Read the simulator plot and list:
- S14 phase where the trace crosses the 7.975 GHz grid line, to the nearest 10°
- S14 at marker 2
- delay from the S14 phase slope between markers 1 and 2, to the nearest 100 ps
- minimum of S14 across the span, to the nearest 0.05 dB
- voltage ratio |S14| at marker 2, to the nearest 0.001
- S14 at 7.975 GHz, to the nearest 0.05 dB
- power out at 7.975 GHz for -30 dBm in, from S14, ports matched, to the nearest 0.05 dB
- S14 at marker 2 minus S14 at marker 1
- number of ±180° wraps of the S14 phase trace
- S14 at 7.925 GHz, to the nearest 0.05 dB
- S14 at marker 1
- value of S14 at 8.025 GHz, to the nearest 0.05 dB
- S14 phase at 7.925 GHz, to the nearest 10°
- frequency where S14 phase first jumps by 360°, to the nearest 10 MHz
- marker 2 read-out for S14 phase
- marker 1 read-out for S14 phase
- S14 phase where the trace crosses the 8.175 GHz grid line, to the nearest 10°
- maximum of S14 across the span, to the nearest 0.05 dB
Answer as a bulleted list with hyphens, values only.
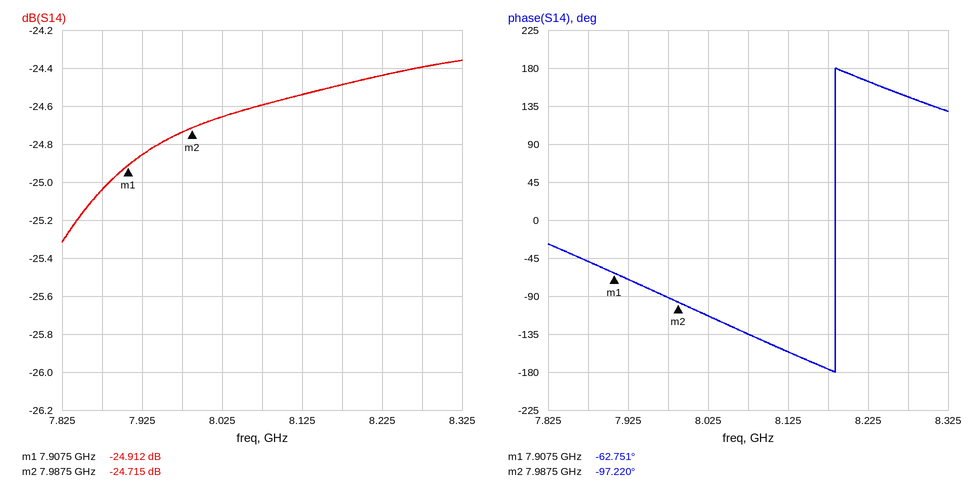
- -90°
- -24.715 dB
- 1.2 ns
- -25.30 dB
- 0.058
- -24.75 dB
- -54.75 dBm
- 0.197 dB
- 1
- -24.85 dB
- -24.912 dB
- -24.65 dB
- -70°
- 8.18 GHz
- -97.220°
- -62.751°
- -180°
- -24.35 dB
